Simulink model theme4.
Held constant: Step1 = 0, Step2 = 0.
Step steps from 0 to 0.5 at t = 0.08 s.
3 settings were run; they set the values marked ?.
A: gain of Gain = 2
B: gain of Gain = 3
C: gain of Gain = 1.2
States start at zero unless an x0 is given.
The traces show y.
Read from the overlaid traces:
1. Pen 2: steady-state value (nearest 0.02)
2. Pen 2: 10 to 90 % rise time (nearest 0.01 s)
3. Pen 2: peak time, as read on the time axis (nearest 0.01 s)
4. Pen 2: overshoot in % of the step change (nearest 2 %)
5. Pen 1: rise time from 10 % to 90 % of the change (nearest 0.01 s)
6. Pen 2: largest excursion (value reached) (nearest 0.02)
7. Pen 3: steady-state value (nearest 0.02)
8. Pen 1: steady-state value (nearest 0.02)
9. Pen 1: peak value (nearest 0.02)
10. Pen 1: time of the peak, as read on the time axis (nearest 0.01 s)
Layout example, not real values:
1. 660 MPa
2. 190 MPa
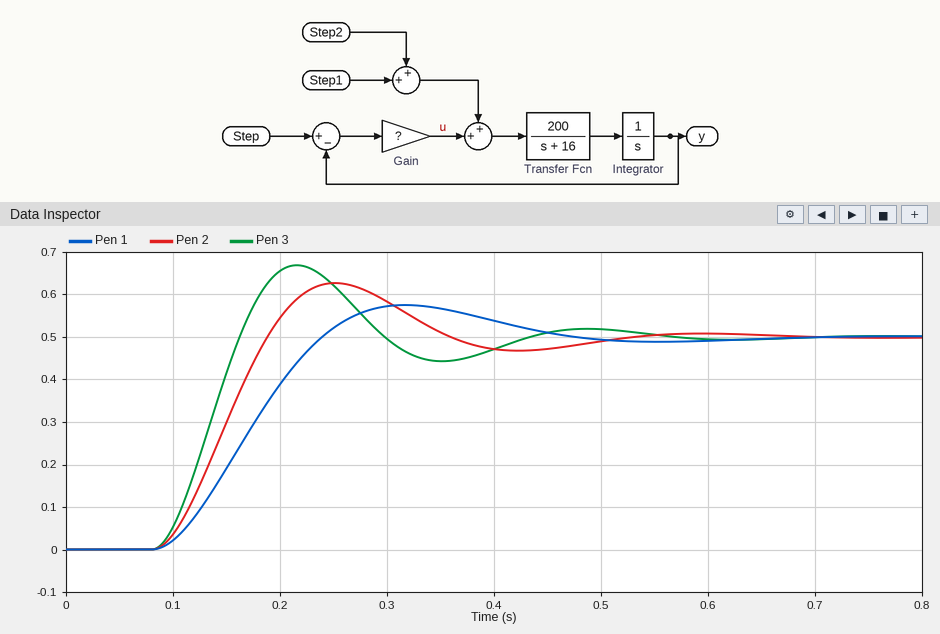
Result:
1. 0.50
2. 0.07 s
3. 0.25 s
4. 26 %
5. 0.11 s
6. 0.62
7. 0.50
8. 0.50
9. 0.58
10. 0.32 s
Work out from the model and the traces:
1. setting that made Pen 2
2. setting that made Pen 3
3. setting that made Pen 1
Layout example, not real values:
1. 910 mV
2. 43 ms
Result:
1. A
2. B
3. C
